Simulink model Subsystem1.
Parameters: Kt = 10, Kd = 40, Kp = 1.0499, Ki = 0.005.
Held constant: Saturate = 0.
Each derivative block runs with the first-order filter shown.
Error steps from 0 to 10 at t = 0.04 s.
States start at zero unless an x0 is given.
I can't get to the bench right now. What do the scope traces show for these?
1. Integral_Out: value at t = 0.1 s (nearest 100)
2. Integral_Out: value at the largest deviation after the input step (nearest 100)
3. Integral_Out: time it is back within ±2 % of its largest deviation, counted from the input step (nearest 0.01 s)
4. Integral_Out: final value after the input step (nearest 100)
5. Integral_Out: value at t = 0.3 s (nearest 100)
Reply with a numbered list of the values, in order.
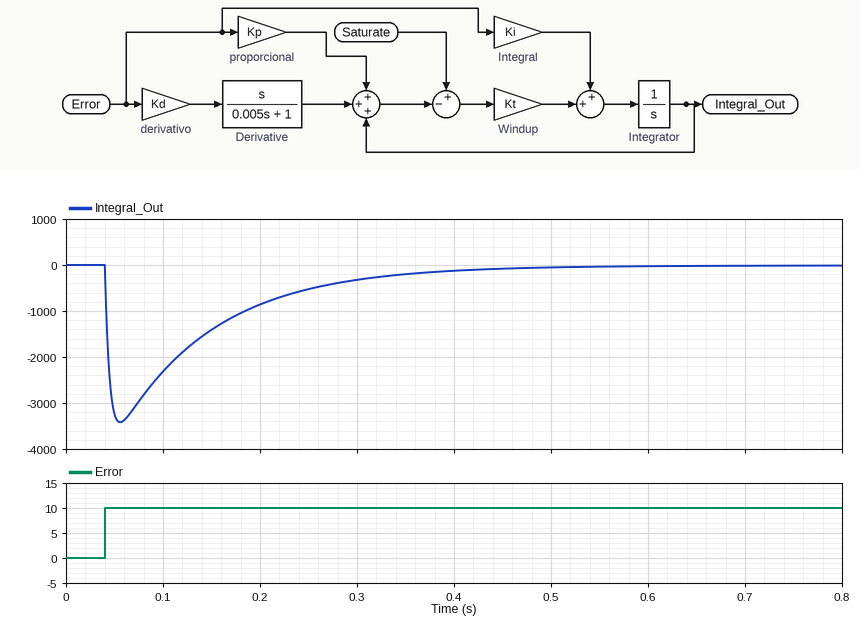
1. -2300
2. -3400
3. 0.41 s
4. 0
5. -300
